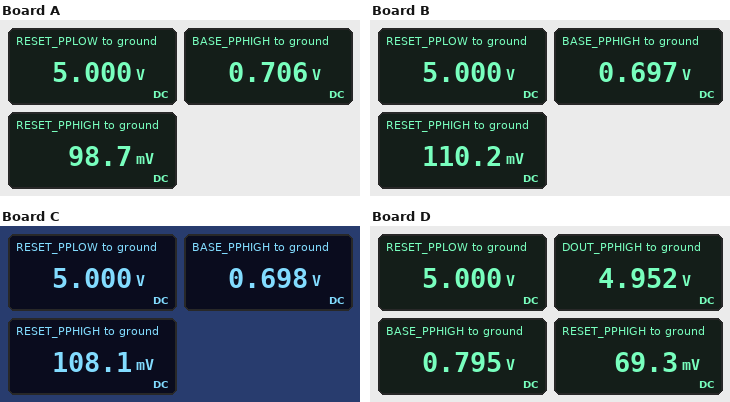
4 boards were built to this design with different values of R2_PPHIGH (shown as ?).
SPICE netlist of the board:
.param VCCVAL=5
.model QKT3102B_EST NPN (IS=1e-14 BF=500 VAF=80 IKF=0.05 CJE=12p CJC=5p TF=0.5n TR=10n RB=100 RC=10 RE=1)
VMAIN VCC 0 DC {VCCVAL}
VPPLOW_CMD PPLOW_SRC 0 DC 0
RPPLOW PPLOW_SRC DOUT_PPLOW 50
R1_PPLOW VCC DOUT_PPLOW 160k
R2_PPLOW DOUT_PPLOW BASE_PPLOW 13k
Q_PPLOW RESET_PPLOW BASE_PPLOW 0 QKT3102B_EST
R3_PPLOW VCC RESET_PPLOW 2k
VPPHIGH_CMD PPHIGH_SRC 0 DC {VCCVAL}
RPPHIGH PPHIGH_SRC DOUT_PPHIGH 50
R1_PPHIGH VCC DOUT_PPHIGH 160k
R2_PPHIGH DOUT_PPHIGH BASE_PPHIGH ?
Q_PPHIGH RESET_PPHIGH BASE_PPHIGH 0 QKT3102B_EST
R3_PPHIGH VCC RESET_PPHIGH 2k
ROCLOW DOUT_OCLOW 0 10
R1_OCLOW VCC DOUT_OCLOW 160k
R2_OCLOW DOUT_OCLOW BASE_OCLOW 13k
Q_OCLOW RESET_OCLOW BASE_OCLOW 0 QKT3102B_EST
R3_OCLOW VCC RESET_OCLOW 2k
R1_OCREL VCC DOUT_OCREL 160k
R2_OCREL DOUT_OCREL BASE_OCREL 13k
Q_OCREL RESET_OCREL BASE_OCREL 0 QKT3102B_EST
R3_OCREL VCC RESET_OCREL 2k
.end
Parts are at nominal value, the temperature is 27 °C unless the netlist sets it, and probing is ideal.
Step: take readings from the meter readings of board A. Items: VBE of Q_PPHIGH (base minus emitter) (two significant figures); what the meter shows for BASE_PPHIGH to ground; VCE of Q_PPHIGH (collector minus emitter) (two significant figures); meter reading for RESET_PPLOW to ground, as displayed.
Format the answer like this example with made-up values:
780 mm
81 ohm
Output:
710 mV
0.706 V
99 mV
5.000 V
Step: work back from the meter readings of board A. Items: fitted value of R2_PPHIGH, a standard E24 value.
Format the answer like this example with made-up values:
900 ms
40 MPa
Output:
22 kΩ
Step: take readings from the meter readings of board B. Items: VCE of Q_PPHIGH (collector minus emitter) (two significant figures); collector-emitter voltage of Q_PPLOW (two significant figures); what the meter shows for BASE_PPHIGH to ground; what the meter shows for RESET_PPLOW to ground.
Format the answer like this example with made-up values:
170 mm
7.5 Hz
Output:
110 mV
5.0 V
0.697 V
5.000 V
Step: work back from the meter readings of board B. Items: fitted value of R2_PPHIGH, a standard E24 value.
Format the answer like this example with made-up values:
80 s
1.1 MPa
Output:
36 kΩ
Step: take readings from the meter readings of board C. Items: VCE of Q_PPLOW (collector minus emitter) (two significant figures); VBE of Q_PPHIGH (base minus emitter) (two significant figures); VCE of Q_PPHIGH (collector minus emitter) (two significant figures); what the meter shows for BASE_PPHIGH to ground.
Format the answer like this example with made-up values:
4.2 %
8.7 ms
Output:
5.0 V
700 mV
110 mV
0.698 V
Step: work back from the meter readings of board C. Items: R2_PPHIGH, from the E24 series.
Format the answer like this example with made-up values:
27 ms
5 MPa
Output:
33 kΩ
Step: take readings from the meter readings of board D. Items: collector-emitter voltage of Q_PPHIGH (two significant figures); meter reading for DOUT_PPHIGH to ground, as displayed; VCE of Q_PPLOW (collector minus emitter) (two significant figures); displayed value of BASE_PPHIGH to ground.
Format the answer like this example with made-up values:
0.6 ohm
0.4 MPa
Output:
69 mV
4.952 V
5.0 V
0.795 V
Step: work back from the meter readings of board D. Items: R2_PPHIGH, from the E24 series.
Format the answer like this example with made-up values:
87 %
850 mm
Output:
4.3 kΩ
